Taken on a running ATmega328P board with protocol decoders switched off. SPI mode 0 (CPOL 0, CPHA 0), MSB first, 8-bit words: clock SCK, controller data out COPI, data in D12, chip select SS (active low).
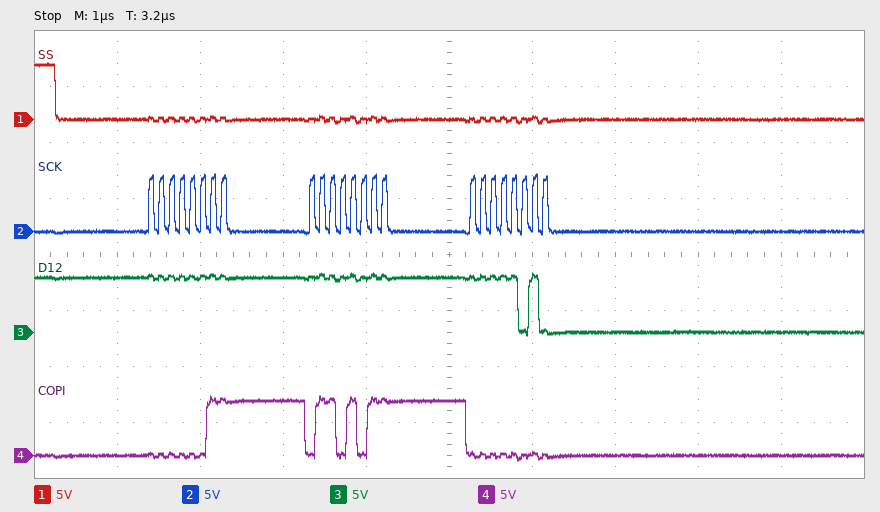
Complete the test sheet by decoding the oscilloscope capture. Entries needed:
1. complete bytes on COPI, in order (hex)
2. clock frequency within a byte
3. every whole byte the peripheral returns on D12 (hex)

03 6B 00
8 MHz
FF FF FA
